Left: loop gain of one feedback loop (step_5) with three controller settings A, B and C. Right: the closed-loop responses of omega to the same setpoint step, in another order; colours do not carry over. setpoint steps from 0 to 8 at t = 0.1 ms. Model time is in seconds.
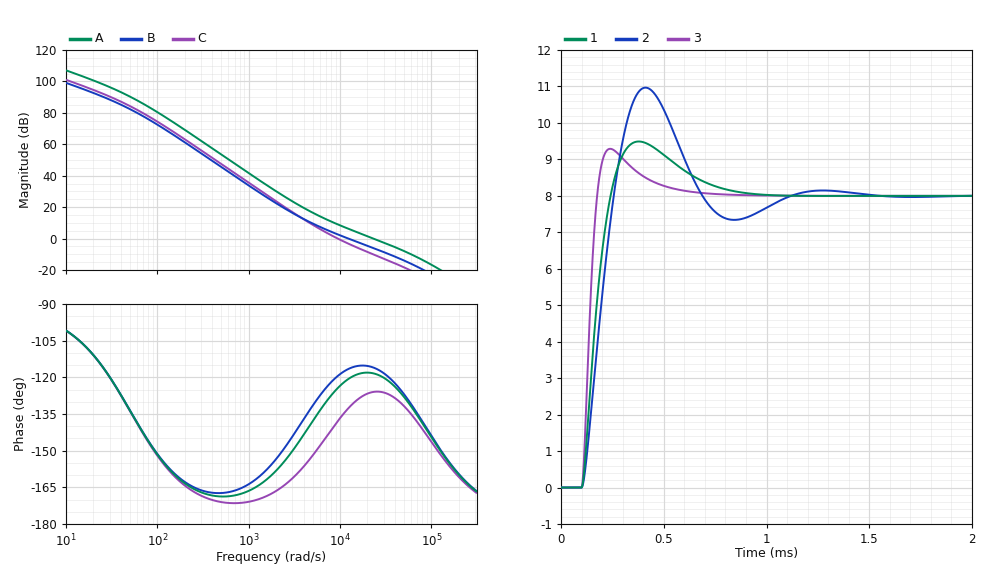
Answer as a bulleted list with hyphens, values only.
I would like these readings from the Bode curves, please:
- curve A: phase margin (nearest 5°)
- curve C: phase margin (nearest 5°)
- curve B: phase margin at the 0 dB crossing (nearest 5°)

- 60°
- 40°
- 65°
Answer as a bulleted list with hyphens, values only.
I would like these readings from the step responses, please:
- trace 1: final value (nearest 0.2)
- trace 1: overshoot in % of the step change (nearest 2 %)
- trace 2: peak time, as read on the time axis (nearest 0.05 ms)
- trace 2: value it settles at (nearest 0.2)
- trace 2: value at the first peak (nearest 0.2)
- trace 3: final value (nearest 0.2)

- 8.0
- 18 %
- 0.40 ms
- 8.0
- 11.0
- 8.0
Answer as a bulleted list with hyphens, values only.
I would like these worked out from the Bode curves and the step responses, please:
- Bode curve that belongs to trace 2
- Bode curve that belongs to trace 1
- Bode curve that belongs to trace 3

- C
- B
- A
